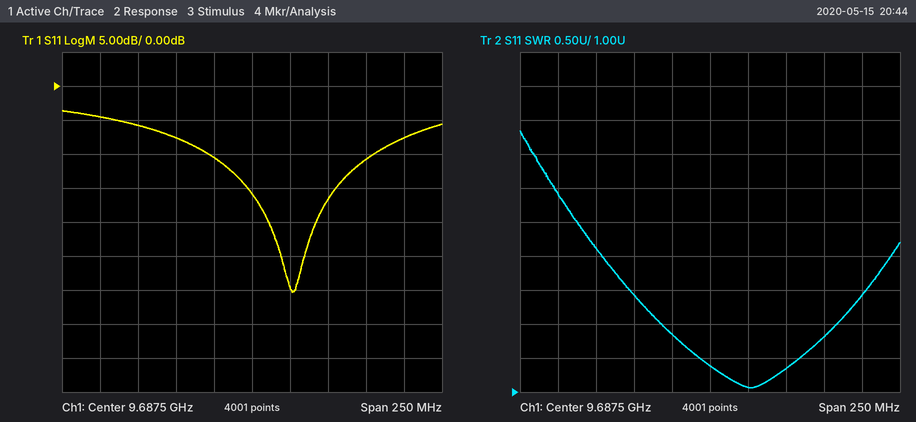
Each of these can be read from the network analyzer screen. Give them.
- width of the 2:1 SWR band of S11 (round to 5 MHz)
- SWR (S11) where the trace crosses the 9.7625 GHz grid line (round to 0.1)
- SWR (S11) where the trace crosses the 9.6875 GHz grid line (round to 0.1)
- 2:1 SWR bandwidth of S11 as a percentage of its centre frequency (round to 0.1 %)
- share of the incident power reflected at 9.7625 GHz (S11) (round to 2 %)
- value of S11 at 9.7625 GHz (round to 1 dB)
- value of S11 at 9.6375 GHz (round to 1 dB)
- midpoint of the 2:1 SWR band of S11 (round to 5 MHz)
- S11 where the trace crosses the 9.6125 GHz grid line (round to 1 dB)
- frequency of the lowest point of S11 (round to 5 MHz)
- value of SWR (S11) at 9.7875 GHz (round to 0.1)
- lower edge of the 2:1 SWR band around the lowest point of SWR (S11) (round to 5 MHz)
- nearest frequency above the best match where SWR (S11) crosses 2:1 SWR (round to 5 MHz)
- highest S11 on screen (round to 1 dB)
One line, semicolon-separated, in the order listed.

115 MHz; 1.8; 1.4; 1.2 %; 8 %; -11 dB; -8 dB; 9.715 GHz; -6 dB; 9.715 GHz; 2.4; 9.655 GHz; 9.770 GHz; -4 dB
